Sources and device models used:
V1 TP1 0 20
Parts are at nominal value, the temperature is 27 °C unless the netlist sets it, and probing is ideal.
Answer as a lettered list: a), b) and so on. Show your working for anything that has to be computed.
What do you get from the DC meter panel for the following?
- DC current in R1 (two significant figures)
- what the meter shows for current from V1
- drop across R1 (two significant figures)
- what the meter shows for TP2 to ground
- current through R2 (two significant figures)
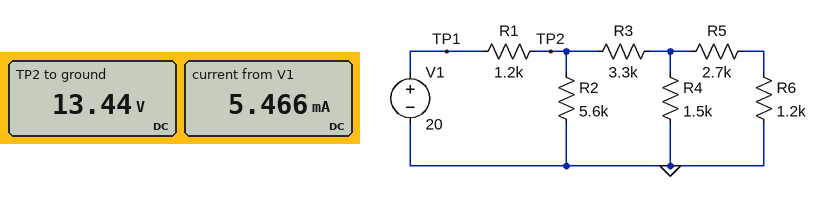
a) (20 V - 13.44 V) / 1.2 kΩ = 5.5 mA
b) 5.466 mA
c) 20 V - 13.44 V = 6.6 V
d) 13.44 V
e) (13.44 V) / 5.6 kΩ = 2.4 mA
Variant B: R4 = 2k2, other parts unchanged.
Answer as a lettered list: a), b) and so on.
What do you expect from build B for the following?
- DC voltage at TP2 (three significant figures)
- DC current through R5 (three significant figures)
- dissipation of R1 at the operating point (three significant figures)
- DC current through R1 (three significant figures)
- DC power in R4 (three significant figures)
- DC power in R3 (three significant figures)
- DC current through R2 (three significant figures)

a) 13.6 V
b) 1.04 mA
c) 34.0 mW
d) 5.32 mA
e) 7.52 mW
f) 27.6 mW
g) 2.43 mA
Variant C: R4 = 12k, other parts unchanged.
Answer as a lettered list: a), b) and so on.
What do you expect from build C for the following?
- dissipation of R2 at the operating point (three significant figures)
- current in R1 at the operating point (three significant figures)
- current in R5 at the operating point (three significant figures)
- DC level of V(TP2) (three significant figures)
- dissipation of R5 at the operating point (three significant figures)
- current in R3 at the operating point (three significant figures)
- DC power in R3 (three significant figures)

a) 36.1 mW
b) 4.82 mA
c) 1.72 mA
d) 14.2 V
e) 7.98 mW
f) 2.28 mA
g) 17.1 mW
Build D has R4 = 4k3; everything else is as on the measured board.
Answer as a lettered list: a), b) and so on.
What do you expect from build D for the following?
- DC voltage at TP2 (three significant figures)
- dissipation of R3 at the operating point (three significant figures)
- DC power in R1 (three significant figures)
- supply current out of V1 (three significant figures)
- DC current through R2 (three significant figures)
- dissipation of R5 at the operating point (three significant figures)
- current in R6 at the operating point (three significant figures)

a) 13.9 V
b) 22.3 mW
c) 31.0 mW
d) 5.08 mA
e) 2.48 mA
f) 5.02 mW
g) 1.36 mA
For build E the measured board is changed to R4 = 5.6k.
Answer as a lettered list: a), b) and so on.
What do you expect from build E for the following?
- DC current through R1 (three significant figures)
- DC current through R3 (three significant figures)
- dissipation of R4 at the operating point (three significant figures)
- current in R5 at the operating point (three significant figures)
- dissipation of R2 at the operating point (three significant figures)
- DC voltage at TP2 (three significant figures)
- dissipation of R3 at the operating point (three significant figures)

a) 5.00 mA
b) 2.50 mA
c) 5.90 mW
d) 1.47 mA
e) 35.0 mW
f) 14.0 V
g) 20.6 mW
